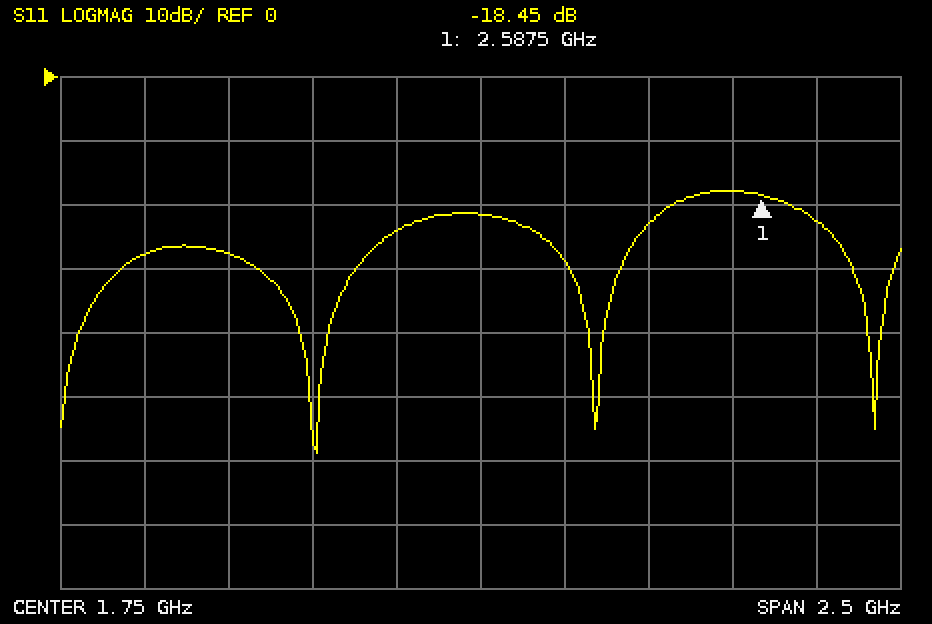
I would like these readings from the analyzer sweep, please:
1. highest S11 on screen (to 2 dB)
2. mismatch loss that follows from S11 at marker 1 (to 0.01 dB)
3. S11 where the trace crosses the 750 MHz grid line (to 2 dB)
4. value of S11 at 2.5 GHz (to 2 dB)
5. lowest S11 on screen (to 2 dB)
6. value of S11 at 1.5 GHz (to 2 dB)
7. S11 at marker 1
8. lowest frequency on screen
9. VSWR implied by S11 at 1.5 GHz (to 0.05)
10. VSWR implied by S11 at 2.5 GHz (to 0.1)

-18 dB
0.06 dB
-28 dB
-18 dB
-58 dB
-24 dB
-18.45 dB
500 MHz
1.15
1.3
